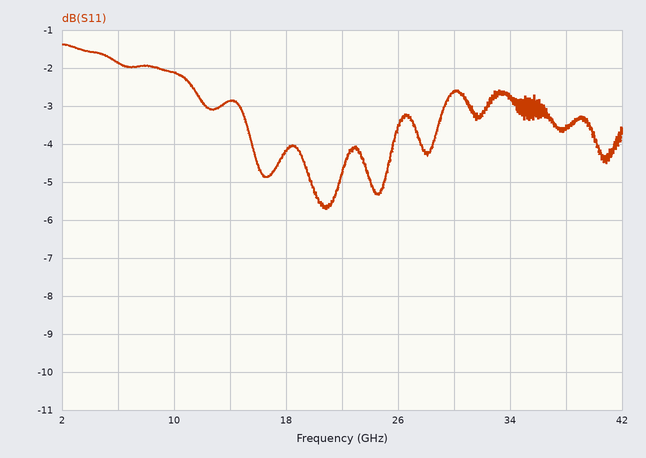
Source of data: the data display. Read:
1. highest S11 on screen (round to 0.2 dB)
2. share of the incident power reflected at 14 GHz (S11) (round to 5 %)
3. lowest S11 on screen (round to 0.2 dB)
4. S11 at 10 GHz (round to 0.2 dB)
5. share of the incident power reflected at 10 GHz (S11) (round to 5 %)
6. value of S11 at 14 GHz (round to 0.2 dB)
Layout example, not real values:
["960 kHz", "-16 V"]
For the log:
["-1.4 dB", "50 %", "-5.8 dB", "-2.2 dB", "60 %", "-2.8 dB"]
